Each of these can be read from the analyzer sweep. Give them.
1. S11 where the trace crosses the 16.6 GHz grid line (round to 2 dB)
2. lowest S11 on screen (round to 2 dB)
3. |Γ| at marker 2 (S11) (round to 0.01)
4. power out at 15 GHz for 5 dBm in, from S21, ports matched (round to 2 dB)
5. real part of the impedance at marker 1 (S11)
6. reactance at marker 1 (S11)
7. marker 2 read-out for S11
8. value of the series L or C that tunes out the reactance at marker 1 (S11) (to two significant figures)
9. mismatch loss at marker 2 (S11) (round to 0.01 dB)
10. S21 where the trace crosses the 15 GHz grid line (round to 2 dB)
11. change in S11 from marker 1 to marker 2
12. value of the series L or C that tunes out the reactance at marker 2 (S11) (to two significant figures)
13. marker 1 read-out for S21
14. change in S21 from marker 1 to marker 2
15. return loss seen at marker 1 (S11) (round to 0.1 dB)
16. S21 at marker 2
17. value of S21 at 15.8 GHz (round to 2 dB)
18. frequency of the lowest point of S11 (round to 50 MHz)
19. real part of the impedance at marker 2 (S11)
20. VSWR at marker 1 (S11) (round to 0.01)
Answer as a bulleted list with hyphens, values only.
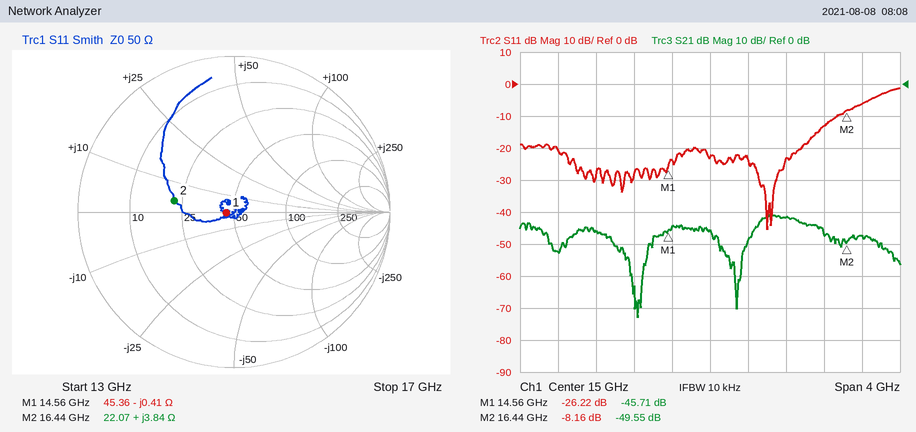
- -6 dB
- -46 dB
- 0.39
- -40 dBm
- 45.36 Ω
- -0.41 Ω
- -8.16 dB
- 4.5 pH
- 0.72 dB
- -46 dB
- 18.06 dB
- 2.5 pF
- -45.71 dB
- -3.84 dB
- 26.2 dB
- -49.55 dB
- -42 dB
- 15.60 GHz
- 22.07 Ω
- 1.10
